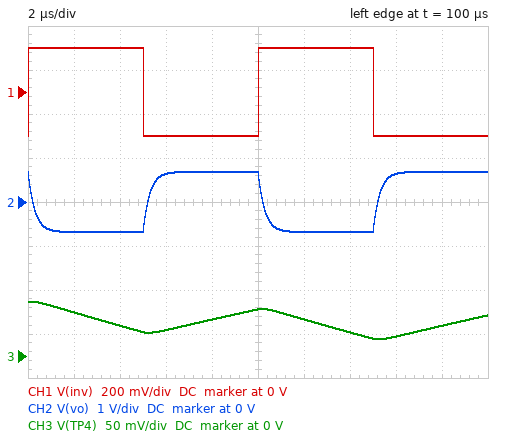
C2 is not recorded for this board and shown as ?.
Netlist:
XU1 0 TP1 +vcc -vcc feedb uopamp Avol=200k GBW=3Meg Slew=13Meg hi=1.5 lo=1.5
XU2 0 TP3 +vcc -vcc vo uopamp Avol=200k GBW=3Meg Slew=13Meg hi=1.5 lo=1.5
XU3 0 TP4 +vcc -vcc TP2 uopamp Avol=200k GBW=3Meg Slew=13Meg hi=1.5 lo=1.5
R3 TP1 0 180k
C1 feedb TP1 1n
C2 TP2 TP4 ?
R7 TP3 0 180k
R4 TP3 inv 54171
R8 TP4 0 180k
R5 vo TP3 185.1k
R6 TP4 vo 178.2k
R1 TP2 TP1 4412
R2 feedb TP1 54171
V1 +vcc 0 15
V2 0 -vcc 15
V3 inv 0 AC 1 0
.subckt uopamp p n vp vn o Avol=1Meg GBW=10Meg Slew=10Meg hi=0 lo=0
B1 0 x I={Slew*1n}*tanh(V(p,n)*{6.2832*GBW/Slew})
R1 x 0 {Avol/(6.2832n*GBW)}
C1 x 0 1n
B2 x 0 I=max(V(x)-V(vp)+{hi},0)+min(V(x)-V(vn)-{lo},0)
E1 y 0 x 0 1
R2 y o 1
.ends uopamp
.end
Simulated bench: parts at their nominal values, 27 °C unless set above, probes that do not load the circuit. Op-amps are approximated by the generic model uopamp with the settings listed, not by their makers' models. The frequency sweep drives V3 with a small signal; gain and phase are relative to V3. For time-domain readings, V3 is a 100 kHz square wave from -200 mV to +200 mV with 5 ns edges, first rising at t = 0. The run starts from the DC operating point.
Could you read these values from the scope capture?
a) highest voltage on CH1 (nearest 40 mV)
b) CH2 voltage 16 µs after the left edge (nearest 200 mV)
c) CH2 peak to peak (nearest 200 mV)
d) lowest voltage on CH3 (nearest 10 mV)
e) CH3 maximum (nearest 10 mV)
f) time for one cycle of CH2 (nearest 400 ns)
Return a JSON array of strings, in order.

["200 mV", "600 mV", "1.4 V", "20 mV", "60 mV", "10.0 µs"]
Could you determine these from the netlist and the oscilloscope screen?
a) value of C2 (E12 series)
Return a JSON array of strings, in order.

["560 pF"]
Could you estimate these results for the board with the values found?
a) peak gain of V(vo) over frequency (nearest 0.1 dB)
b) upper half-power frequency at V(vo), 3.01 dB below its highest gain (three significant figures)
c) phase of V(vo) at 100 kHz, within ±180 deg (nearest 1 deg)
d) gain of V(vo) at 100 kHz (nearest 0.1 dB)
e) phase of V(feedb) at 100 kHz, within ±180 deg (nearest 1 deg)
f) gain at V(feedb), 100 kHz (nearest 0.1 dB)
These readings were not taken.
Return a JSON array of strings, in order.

["10.7 dB", "551 kHz", "170 deg", "10.5 dB", "-12 deg", "-34.4 dB"]
